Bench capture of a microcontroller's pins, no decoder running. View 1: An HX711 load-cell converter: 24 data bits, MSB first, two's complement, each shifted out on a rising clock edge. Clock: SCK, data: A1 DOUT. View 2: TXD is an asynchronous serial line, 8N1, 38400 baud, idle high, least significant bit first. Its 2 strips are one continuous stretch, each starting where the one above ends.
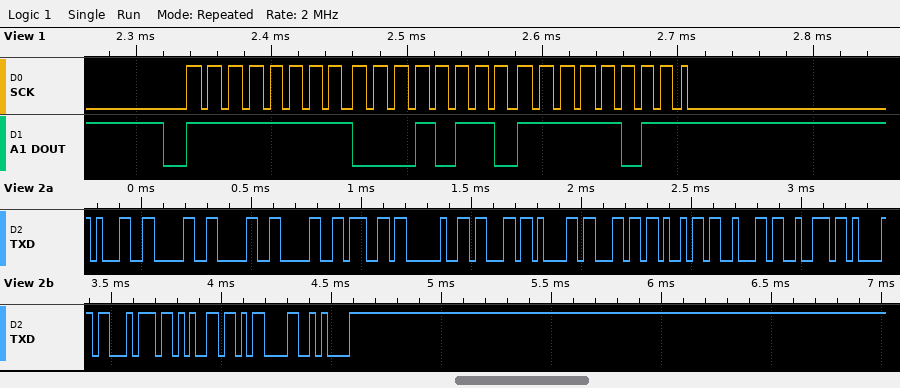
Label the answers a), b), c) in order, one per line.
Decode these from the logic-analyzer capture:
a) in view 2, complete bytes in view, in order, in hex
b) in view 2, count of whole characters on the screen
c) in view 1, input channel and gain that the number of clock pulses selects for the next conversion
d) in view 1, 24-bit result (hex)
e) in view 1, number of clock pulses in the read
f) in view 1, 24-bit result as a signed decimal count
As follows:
a) 0x31 0x30 0x30 0x30 0x67 0x20 0x63 0x61 0x6C 0x69 0x62 0x72 0x61 0x74 0x65 0x0D 0x0A
b) 17
c) channel A, gain 128
d) 0xFF16FB
e) 25
f) -59653
